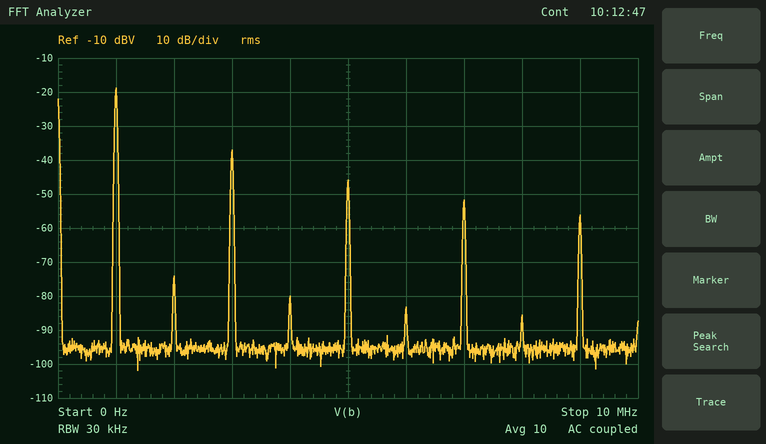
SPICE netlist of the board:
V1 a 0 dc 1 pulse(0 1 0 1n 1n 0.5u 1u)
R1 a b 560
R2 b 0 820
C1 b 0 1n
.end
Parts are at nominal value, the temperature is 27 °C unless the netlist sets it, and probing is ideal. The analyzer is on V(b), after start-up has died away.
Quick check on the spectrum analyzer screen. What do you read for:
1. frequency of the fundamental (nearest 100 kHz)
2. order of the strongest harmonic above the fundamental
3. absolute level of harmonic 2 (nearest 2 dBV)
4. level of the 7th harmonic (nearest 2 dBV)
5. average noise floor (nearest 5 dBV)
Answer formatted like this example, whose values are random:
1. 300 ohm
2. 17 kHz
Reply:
1. 1.0 MHz
2. 3
3. -74 dBV
4. -52 dBV
5. -95 dBV
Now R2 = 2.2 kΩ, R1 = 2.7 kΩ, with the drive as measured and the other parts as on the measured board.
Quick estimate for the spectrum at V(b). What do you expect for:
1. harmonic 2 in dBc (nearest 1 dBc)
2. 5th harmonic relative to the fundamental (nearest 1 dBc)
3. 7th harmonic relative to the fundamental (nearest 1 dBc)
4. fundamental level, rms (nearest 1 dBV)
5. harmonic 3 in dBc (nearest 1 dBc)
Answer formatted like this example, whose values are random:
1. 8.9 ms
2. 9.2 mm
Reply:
1. -56 dBc
2. -28 dBc
3. -34 dBc
4. -32 dBV
5. -19 dBc
